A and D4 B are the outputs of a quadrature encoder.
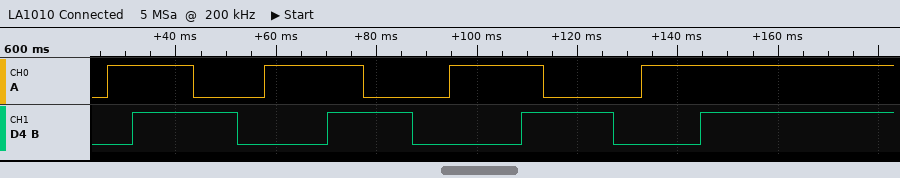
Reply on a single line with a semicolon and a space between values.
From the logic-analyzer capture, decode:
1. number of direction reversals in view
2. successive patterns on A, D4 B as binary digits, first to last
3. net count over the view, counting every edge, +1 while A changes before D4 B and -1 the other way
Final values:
0; 00 10 11 01 00 10 11 01 00 10 11 01 00 10 11; +14
